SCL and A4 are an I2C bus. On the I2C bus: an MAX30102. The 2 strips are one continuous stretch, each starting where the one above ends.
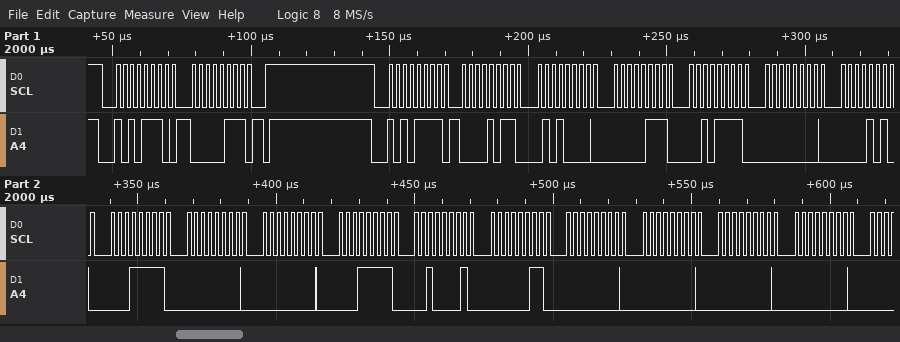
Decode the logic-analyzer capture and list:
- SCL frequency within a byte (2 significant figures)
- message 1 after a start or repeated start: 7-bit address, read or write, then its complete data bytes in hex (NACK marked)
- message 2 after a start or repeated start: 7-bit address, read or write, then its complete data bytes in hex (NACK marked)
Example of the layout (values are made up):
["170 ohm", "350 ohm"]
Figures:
["400 kHz", "0x57 write: 07", "0x57 read: 0B 50 07 2F 00 0A 1F 00 00 1F 21 03 00 00 00 00"]
